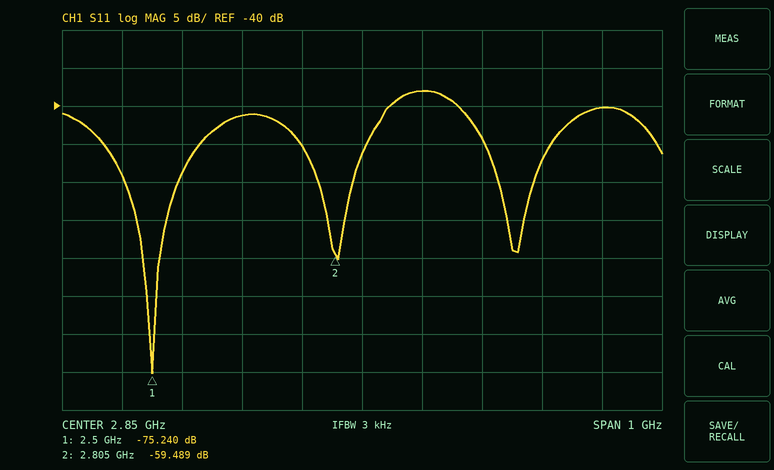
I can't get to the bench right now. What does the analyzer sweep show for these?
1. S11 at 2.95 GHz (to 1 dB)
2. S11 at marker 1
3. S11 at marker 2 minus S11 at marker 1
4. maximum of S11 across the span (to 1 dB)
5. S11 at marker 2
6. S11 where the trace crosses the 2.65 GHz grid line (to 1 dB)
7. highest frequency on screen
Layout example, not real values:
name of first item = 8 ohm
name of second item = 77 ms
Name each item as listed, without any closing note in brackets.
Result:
S11 at 2.95 GHz = -38 dB
S11 at marker 1 = -75.240 dB
S11 at marker 2 minus S11 at marker 1 = 15.751 dB
maximum of S11 across the span = -38 dB
S11 at marker 2 = -59.489 dB
S11 where the trace crosses the 2.65 GHz grid line = -41 dB
highest frequency on screen = 3.35 GHz
